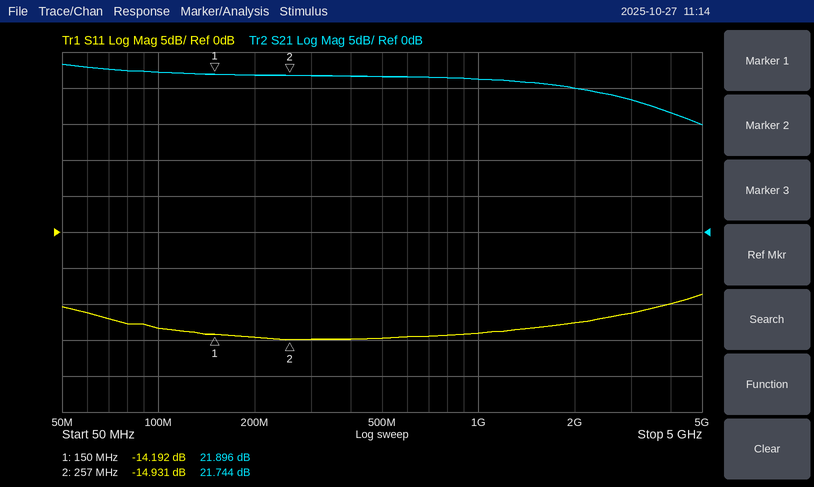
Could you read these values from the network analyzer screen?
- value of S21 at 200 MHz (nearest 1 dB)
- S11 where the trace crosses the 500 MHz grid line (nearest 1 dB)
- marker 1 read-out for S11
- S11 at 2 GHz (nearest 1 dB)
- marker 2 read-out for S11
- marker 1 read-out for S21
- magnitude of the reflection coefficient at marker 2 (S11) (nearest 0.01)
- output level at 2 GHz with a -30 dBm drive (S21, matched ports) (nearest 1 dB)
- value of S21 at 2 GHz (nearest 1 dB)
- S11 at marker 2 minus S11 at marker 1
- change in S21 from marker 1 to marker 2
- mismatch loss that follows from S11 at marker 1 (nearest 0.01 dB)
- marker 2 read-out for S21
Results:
22 dB
-15 dB
-14.192 dB
-13 dB
-14.931 dB
21.896 dB
0.18
-10 dBm
20 dB
-0.739 dB
-0.152 dB
0.17 dB
21.744 dB
